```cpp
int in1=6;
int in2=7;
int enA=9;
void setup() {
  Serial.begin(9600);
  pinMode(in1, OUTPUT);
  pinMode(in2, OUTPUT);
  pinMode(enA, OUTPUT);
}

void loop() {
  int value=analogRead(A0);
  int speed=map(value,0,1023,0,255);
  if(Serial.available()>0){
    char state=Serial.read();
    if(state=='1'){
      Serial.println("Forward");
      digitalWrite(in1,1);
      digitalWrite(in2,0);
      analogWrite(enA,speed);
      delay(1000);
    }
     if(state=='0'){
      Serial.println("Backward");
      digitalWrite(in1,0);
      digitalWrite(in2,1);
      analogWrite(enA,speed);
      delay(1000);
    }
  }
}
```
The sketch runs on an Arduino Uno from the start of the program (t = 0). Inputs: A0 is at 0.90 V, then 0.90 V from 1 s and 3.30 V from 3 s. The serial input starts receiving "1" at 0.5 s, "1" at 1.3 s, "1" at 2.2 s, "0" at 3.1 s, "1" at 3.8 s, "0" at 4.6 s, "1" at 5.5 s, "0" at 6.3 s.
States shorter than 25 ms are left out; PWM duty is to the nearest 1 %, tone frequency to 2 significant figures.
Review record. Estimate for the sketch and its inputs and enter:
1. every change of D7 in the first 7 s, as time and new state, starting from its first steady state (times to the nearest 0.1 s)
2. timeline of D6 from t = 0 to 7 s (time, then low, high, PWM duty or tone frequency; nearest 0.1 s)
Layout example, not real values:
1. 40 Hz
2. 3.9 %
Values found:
1. 0 s low; 3.5 s high; 4.5 s low; 5.5 s high; 6.5 s low
2. 0 s low; 0.5 s high; 3.5 s low; 4.5 s high; 5.5 s low; 6.5 s high
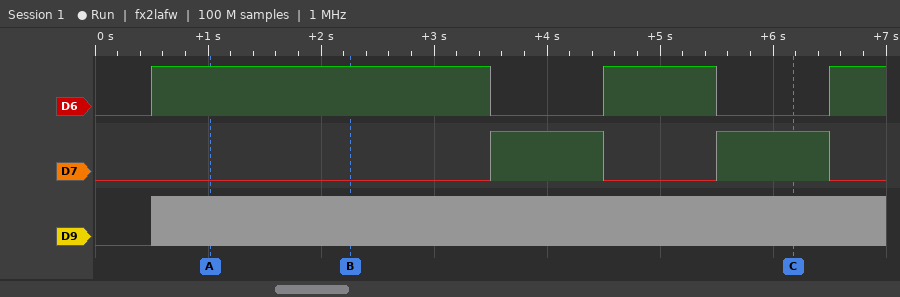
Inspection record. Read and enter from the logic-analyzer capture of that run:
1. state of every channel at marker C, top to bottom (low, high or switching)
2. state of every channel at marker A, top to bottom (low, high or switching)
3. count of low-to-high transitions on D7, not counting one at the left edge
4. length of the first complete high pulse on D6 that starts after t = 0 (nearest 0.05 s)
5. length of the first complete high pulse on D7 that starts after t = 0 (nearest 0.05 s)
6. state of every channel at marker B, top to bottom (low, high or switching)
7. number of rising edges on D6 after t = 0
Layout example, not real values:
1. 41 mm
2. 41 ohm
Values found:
1. D6 low, D7 high, D9 switching
2. D6 high, D7 low, D9 switching
3. 2
4. 3.00 s
5. 1.00 s
6. D6 high, D7 low, D9 switching
7. 3
